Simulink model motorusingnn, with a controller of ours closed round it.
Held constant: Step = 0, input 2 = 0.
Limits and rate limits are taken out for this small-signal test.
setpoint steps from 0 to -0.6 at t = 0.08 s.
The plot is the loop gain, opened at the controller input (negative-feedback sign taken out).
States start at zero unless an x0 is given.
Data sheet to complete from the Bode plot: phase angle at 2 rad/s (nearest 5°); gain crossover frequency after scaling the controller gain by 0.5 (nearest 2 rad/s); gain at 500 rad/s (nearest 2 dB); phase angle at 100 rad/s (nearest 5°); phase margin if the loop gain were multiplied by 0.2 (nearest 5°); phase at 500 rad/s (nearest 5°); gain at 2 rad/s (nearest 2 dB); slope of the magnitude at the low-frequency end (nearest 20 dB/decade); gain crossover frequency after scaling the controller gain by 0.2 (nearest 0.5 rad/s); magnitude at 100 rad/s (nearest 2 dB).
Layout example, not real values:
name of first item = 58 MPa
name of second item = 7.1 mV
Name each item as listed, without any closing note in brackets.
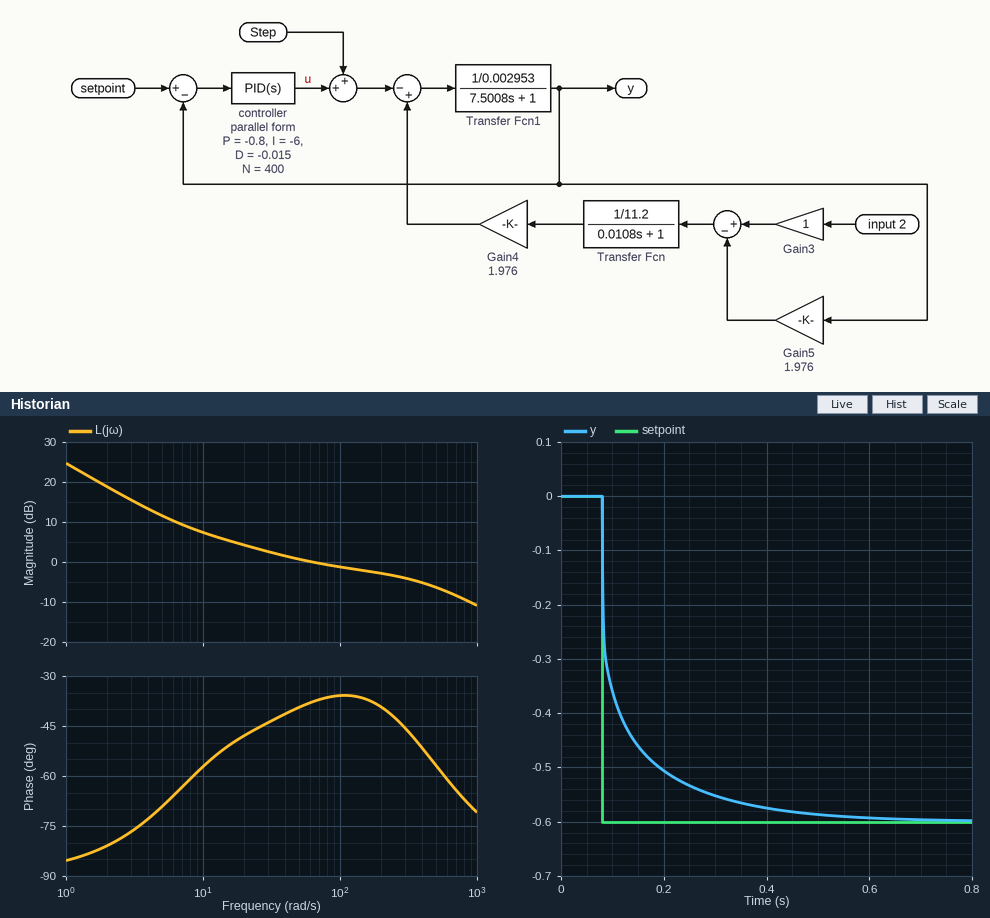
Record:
phase angle at 2 rad/s = -80°
gain crossover frequency after scaling the controller gain by 0.5 = 14 rad/s
gain at 500 rad/s = -6 dB
phase angle at 100 rad/s = -35°
phase margin if the loop gain were multiplied by 0.2 = 105°
phase at 500 rad/s = -55°
gain at 2 rad/s = 18 dB
slope of the magnitude at the low-frequency end = -20 dB/decade
gain crossover frequency after scaling the controller gain by 0.2 = 3.5 rad/s
magnitude at 100 rad/s = -2 dB
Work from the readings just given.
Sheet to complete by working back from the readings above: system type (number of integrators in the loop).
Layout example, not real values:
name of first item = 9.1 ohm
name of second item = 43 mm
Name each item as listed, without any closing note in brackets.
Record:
system type = 1
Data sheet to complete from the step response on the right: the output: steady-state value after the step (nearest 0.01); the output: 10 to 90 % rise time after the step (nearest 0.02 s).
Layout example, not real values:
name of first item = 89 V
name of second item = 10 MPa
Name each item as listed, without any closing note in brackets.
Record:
the output: steady-state value after the step = -0.60
the output: 10 to 90 % rise time after the step = 0.18 s
